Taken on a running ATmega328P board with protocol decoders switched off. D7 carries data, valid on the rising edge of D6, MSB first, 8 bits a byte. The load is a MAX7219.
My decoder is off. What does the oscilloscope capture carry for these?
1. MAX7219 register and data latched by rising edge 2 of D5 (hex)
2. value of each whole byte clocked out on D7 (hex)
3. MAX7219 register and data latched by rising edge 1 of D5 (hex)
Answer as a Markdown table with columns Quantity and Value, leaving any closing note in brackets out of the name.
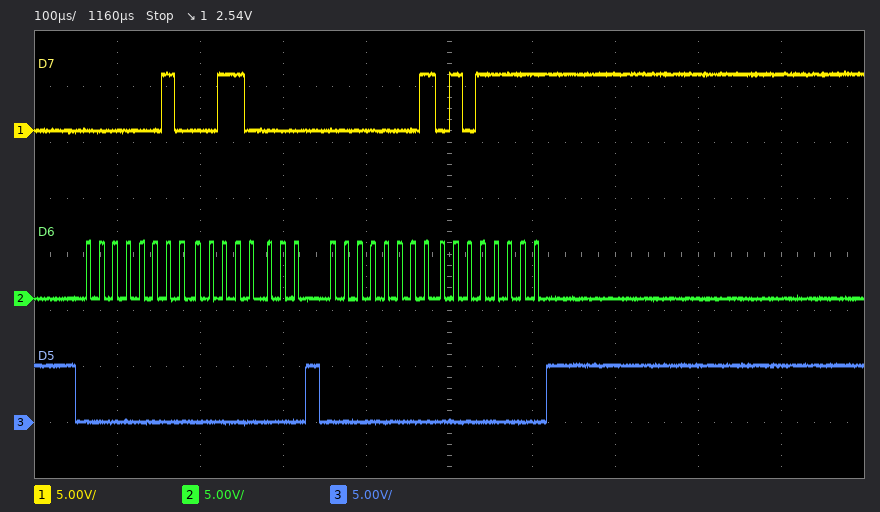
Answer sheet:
| Quantity | Value |
|---|---|
| MAX7219 register and data latched by rising edge 2 of D5 | register 0x1, data 0x5F |
| value of each whole byte clocked out on D7 | 02 30 01 5F |
| MAX7219 register and data latched by rising edge 1 of D5 | register 0x2, data 0x30 |
